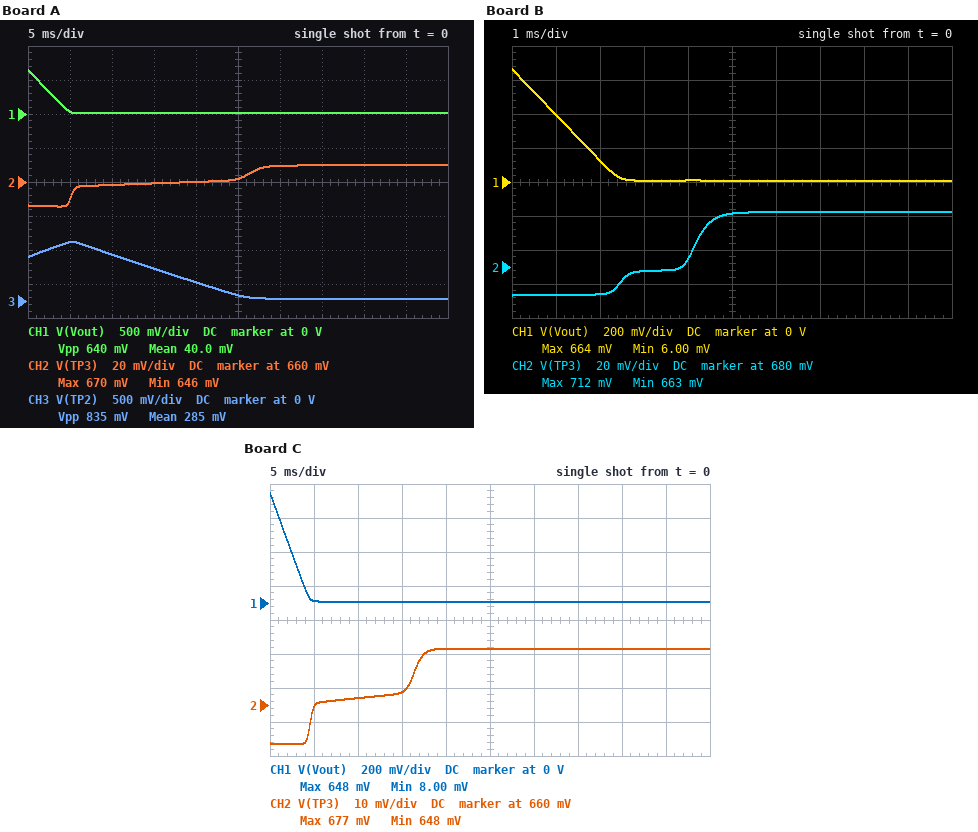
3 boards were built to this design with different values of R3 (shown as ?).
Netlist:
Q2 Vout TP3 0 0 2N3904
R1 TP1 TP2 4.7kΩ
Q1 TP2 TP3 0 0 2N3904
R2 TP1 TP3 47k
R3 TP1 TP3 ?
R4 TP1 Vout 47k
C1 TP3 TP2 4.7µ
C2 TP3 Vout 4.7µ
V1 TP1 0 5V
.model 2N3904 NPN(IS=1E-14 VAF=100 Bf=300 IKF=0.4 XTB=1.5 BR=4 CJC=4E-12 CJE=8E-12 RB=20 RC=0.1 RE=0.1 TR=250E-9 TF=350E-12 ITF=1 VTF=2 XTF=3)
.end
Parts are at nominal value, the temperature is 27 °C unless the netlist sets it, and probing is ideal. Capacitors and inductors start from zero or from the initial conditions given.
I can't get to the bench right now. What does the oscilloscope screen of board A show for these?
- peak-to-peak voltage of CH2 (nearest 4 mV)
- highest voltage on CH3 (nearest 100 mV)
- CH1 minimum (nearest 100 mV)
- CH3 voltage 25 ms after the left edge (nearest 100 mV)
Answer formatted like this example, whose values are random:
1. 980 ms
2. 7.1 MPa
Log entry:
1. 24 mV
2. 900 mV
3. 0 V
4. 100 mV
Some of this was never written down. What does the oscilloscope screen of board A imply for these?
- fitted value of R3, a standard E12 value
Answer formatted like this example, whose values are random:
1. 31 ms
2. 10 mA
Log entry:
1. 15 kΩ
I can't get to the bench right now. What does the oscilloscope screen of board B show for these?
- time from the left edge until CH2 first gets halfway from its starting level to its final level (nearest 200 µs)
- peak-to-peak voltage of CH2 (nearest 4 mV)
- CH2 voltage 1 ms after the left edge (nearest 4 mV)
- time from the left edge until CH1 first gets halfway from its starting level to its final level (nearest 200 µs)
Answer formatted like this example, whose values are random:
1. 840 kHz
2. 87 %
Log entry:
1. 4.0 ms
2. 48 mV
3. 664 mV
4. 1.2 ms
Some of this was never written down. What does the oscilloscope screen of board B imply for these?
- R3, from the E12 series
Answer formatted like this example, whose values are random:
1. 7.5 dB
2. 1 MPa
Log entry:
1. 2.7 kΩ
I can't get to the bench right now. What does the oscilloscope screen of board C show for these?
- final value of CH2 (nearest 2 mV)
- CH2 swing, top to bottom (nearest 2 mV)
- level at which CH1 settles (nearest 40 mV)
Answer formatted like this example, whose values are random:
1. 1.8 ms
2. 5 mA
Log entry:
1. 676 mV
2. 28 mV
3. 0 V
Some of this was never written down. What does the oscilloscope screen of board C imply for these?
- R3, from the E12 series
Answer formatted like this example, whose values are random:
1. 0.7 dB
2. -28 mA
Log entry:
1. 10 kΩ
